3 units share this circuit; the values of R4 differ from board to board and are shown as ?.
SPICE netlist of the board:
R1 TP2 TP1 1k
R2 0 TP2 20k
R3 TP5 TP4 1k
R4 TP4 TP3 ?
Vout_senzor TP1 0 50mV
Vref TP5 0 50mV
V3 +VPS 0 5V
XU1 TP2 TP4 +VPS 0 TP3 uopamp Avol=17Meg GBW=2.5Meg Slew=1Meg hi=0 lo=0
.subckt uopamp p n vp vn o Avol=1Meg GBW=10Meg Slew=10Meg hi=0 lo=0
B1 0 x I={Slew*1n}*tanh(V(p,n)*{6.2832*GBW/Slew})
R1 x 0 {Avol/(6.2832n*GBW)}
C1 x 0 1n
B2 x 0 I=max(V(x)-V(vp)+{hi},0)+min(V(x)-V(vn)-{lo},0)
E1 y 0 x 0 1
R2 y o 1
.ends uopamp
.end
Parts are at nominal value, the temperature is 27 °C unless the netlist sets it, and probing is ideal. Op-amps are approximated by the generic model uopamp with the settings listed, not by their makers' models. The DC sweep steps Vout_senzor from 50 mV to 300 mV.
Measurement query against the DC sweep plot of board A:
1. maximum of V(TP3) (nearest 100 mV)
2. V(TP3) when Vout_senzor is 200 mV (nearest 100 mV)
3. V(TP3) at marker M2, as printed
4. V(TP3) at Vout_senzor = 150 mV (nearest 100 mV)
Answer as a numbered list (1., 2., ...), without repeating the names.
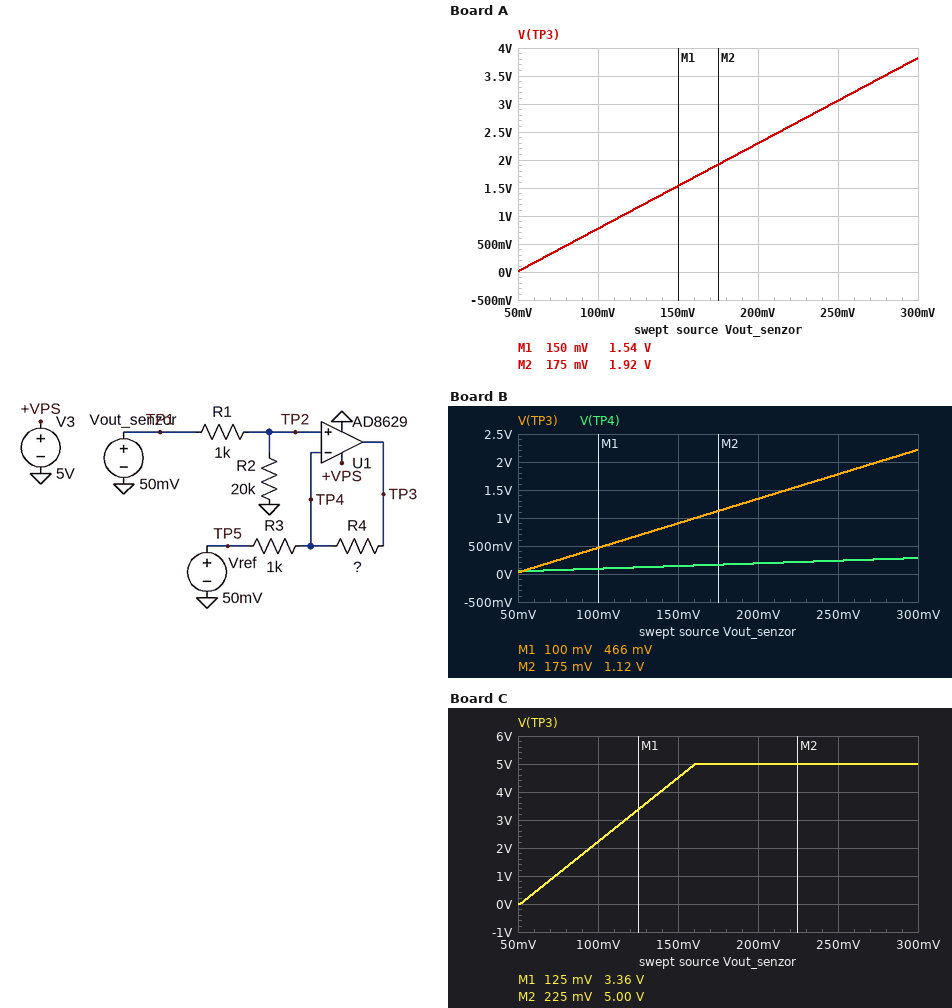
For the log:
1. 3.8 V
2. 2.3 V
3. 1.92 V
4. 1.5 V
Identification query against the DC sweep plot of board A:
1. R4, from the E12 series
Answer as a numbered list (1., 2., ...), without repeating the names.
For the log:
1. 15 kΩ
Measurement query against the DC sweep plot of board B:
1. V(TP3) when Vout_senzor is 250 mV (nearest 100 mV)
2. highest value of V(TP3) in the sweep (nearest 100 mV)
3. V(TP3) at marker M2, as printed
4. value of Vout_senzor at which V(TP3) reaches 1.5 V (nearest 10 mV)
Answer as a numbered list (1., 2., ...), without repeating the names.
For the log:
1. 1.8 V
2. 2.2 V
3. 1.12 V
4. 220 mV
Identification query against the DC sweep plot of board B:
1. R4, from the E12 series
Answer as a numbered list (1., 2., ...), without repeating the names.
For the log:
1. 8.2 kΩ
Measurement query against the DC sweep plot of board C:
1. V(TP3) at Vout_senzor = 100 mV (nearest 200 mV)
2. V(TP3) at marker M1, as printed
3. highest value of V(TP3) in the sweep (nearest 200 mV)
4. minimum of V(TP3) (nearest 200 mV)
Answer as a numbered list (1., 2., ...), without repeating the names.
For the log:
1. 2.2 V
2. 3.36 V
3. 5.0 V
4. 0 V
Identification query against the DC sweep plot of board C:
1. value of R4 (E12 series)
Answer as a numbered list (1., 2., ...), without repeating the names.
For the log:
1. 47 kΩ
